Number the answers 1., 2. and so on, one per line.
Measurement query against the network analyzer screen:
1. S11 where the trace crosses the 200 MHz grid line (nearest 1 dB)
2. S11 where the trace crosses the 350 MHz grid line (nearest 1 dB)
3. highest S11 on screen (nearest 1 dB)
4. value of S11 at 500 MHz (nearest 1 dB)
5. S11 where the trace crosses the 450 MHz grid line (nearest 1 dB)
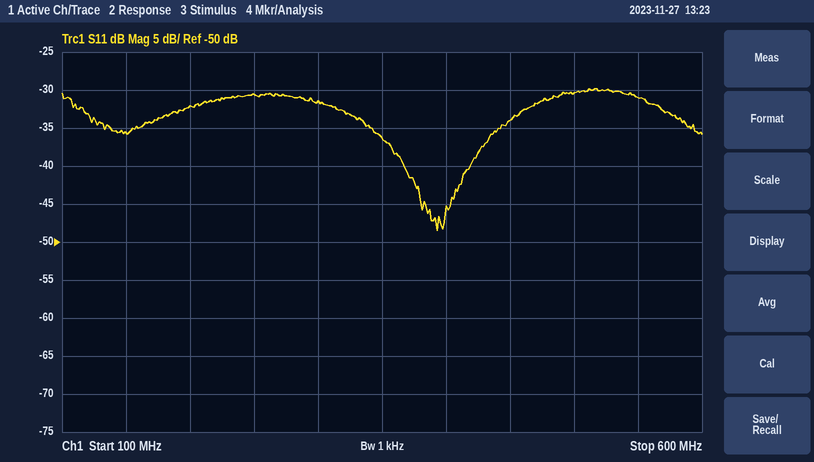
1. -32 dB
2. -36 dB
3. -30 dB
4. -30 dB
5. -34 dB
